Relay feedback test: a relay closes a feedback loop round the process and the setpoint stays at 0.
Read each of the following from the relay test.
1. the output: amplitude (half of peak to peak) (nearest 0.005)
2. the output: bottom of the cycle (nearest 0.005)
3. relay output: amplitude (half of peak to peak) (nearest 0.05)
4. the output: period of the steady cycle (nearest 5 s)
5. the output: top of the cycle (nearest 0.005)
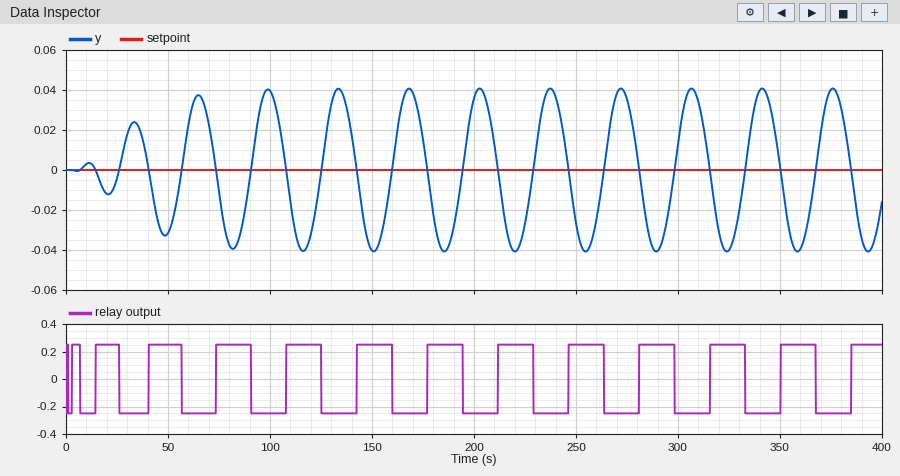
0.040
-0.040
0.25
35 s
0.040
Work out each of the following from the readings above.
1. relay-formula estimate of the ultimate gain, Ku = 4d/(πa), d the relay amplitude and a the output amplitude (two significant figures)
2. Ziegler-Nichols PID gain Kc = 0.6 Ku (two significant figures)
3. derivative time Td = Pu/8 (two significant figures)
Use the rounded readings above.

8.0
4.8
4.4 s
